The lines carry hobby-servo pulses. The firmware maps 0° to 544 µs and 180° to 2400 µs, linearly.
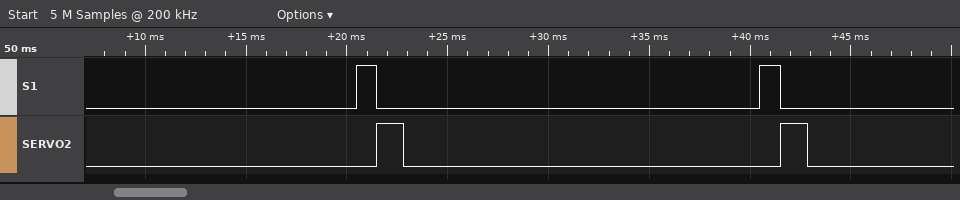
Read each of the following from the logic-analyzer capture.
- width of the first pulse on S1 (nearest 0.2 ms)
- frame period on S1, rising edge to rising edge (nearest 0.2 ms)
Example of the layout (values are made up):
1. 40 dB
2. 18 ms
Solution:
1. 1.0 ms
2. 20.0 ms
